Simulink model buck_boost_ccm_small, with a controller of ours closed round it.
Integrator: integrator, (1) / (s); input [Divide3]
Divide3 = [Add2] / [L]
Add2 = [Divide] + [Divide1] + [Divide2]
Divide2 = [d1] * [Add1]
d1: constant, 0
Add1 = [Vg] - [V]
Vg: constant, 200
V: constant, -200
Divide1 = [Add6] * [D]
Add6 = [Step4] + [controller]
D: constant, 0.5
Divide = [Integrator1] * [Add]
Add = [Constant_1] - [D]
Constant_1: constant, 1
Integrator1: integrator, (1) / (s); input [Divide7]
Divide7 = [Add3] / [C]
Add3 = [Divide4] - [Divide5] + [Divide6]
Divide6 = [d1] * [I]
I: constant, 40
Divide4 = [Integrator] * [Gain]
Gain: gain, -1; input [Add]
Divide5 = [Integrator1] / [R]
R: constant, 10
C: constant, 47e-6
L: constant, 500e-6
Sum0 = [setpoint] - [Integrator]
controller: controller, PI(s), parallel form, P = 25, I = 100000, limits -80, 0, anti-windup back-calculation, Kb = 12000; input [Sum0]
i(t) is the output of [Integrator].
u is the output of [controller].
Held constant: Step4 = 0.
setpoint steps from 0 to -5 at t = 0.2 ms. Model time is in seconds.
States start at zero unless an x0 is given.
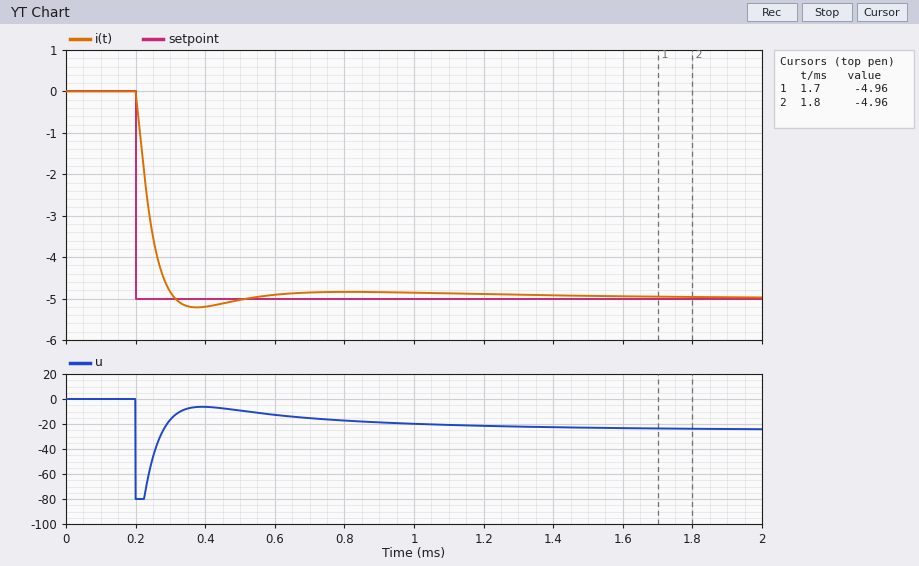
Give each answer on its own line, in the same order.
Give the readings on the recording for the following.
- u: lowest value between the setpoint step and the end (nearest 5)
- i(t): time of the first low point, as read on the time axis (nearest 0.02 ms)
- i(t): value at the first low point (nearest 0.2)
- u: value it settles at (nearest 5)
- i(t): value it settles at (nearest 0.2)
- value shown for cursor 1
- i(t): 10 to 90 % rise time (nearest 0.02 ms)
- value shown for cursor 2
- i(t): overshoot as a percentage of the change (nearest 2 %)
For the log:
-80
0.38 ms
-5.2
-25
-5.0
-4.96
0.08 ms
-4.96
4 %
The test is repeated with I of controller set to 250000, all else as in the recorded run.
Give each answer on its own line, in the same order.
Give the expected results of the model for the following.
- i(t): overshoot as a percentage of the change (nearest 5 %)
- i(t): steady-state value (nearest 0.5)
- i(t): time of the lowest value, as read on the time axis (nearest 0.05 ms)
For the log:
15 %
-5.0
0.35 ms
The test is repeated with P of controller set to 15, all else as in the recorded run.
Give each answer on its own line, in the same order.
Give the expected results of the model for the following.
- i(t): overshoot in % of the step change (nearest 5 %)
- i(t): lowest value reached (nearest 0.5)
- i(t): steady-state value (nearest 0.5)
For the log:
15 %
-5.5
-5.0
